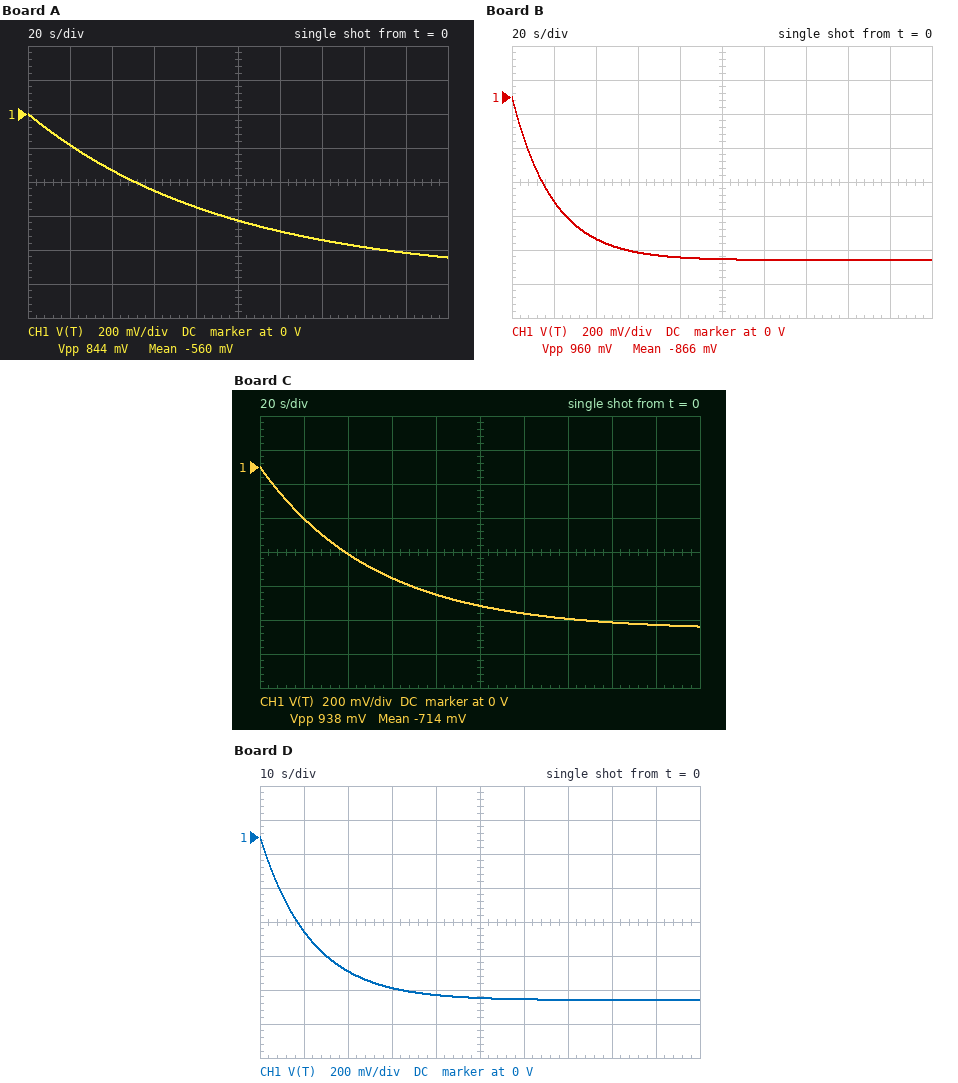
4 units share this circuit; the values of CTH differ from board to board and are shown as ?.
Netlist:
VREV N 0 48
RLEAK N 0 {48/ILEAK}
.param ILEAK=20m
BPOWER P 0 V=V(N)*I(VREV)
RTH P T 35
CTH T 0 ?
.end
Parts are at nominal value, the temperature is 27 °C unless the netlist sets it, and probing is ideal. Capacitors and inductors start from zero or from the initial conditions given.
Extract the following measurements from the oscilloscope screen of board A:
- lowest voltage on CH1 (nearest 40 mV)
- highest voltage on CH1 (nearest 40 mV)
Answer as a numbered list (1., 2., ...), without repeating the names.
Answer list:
1. -840 mV
2. 0 V
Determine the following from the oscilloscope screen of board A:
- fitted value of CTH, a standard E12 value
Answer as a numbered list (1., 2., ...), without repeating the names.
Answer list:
1. 2.7 F
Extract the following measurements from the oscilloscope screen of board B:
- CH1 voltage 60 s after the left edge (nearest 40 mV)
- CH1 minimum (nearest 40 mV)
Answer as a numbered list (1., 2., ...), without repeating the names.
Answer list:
1. -920 mV
2. -960 mV
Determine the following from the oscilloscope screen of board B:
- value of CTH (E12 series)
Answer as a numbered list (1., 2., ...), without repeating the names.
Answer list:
1. 560 mF
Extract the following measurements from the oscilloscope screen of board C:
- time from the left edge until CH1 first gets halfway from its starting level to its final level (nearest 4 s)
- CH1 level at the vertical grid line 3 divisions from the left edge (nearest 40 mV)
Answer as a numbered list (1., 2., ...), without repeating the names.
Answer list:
1. 36 s
2. -640 mV
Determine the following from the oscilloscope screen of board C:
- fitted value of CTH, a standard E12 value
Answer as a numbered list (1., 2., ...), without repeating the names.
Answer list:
1. 1.5 F
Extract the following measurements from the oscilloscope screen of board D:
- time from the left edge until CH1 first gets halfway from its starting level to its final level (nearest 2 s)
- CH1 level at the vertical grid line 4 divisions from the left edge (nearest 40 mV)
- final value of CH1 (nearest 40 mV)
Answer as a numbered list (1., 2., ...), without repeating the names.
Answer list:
1. 8 s
2. -920 mV
3. -960 mV
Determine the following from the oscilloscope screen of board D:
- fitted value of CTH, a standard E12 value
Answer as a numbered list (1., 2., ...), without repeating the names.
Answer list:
1. 330 mF
